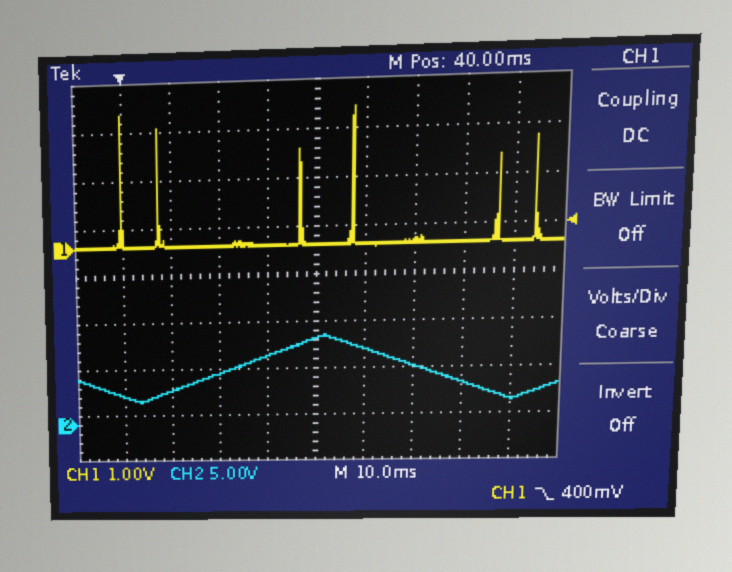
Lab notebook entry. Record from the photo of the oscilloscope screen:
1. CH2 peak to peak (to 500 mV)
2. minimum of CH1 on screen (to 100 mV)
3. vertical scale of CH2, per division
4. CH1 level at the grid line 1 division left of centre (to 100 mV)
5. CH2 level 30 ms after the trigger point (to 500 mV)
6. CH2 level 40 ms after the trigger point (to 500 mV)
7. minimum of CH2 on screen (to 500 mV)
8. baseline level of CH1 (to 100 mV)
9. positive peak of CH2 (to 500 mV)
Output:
7.0 V
0.0 V
5 V
0.0 V
7.5 V
9.0 V
2.5 V
0.0 V
9.5 V
